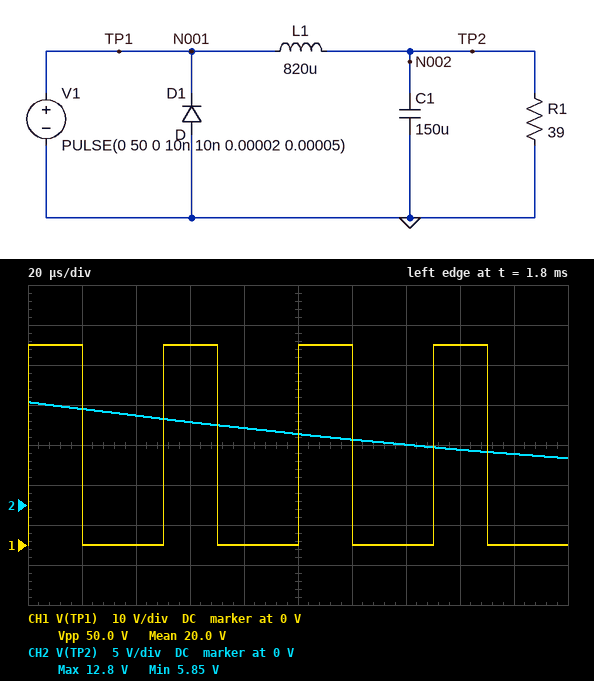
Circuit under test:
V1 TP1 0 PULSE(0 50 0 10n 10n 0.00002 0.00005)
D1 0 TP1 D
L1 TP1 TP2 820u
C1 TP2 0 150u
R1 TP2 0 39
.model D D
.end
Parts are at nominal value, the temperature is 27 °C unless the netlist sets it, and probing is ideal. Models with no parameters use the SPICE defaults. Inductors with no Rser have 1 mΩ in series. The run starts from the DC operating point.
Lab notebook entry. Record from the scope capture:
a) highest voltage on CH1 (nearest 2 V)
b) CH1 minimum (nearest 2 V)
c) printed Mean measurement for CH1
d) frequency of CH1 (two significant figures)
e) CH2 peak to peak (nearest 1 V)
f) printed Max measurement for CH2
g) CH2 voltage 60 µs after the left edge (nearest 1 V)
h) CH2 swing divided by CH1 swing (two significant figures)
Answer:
50 V
0 V
20.0 V
20 kHz
7 V
12.8 V
10 V
0.14
